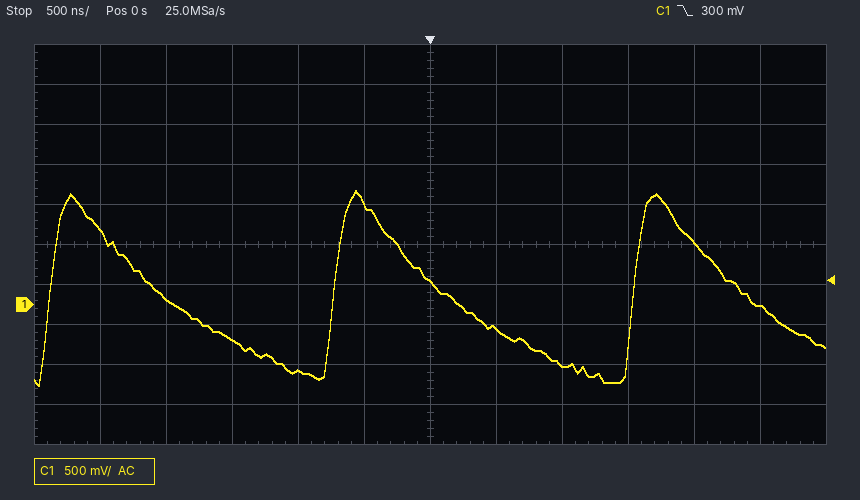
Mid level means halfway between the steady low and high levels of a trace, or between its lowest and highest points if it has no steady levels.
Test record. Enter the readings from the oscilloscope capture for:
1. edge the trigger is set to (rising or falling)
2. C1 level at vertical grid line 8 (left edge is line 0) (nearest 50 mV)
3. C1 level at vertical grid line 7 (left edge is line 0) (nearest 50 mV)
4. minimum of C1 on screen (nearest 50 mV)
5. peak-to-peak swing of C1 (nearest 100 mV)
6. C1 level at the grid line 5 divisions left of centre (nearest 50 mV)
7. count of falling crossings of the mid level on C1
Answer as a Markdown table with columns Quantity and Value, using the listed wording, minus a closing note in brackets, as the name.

| Quantity | Value |
|---|---|
| edge the trigger is set to | falling |
| C1 level at vertical grid line 8 (left edge is line 0) | -750 mV |
| C1 level at vertical grid line 7 (left edge is line 0) | -300 mV |
| minimum of C1 on screen | -1.00 V |
| peak-to-peak swing of C1 | 2.40 V |
| C1 level at the grid line 5 divisions left of centre | 950 mV |
| count of falling crossings of the mid level on C1 | 3 |
